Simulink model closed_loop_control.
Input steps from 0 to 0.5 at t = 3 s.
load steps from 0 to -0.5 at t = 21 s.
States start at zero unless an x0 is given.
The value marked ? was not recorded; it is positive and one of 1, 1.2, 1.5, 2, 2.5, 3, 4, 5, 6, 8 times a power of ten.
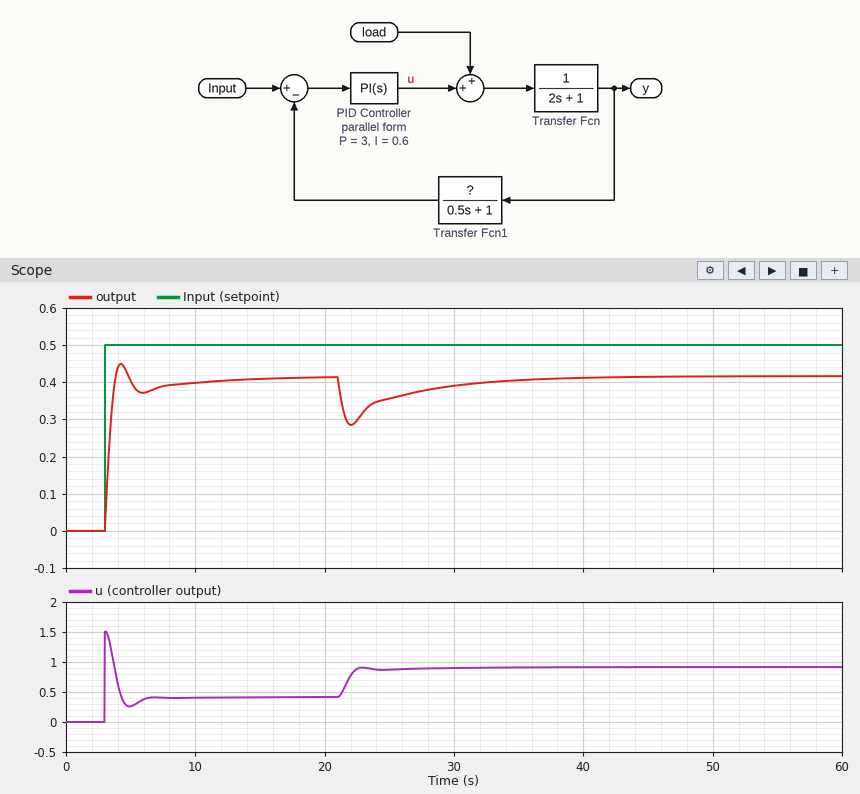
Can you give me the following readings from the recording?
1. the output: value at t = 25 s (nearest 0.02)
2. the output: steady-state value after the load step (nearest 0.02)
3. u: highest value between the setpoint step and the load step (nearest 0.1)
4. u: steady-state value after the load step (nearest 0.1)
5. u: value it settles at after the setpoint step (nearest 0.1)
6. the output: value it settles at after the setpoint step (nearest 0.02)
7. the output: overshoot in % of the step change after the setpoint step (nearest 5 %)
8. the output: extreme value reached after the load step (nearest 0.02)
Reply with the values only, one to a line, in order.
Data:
0.36
0.42
1.5
0.9
0.4
0.42
10 %
0.28
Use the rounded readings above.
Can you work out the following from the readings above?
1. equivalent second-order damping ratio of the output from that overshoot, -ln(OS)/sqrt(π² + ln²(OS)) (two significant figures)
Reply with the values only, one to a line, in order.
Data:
0.59
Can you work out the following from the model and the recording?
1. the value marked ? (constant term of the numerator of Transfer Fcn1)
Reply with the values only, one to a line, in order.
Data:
1.2
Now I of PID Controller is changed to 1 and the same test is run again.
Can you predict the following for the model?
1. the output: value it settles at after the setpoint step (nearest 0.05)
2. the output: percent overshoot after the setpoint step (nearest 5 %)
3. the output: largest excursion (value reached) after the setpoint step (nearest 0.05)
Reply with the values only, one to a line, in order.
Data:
0.40
15 %
0.50
